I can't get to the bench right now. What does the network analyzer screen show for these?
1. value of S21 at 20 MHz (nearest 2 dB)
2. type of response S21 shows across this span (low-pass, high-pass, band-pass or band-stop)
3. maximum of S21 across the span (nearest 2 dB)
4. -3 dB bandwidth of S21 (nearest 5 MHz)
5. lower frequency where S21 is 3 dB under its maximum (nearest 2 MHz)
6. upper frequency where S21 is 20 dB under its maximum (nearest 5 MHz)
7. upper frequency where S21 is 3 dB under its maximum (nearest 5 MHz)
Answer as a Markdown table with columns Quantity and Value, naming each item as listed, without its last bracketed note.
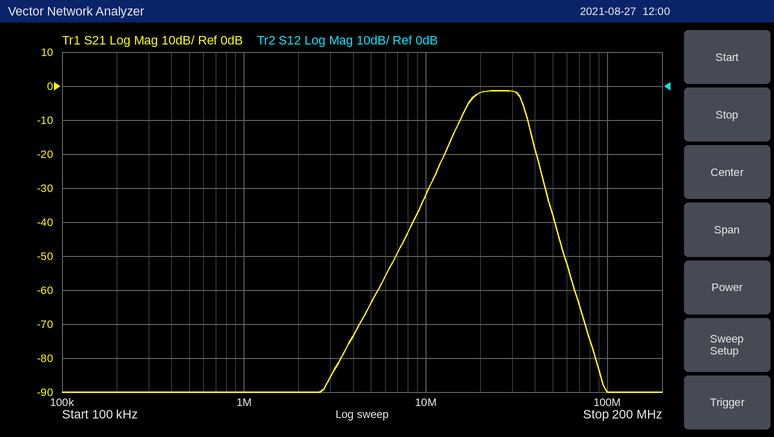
| Quantity | Value |
|---|---|
| value of S21 at 20 MHz | -2 dB |
| type of response S21 shows across this span | band-pass |
| maximum of S21 across the span | -2 dB |
| -3 dB bandwidth of S21 | 15 MHz |
| lower frequency where S21 is 3 dB under its maximum | 18 MHz |
| upper frequency where S21 is 20 dB under its maximum | 40 MHz |
| upper frequency where S21 is 3 dB under its maximum | 35 MHz |
